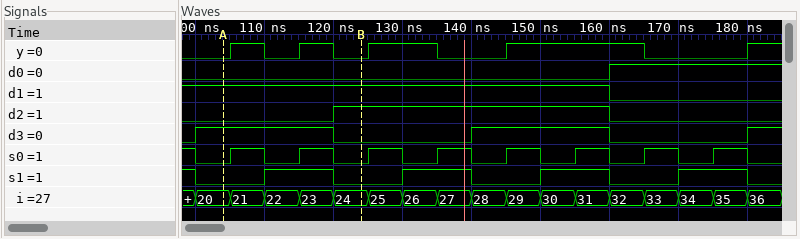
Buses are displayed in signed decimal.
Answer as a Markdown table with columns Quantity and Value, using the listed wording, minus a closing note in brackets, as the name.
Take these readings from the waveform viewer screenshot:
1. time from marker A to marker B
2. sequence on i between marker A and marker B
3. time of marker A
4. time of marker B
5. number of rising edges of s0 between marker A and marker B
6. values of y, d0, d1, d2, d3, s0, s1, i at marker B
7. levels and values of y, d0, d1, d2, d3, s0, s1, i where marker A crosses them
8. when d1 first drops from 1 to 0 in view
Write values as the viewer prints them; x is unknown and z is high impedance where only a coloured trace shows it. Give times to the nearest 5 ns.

| Quantity | Value |
|---|---|
| time from marker A to marker B | 20 ns |
| sequence on i between marker A and marker B | 20, 21, 22, 23, 24 |
| time of marker A | 105 ns |
| time of marker B | 125 ns |
| number of rising edges of s0 between marker A and marker B | 2 |
| values of y, d0, d1, d2, d3, s0, s1, i at marker B | y=0, d0=0, d1=1, d2=1, d3=0, s0=0, s1=0, i=24 |
| levels and values of y, d0, d1, d2, d3, s0, s1, i where marker A crosses them | y=0, d0=0, d1=1, d2=0, d3=1, s0=0, s1=0, i=20 |
| when d1 first drops from 1 to 0 in view | 160 ns |
